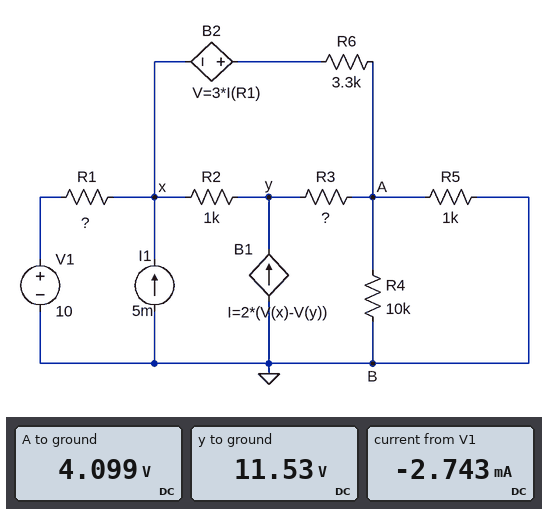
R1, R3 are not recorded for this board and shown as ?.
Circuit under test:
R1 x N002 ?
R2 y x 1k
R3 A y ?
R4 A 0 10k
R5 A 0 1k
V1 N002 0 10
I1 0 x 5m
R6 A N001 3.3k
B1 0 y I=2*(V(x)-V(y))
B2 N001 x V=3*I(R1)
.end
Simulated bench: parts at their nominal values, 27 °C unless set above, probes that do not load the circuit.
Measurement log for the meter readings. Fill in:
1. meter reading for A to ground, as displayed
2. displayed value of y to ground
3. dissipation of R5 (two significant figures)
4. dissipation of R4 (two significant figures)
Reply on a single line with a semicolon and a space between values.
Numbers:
4.099 V; 11.53 V; 17 mW; 1.7 mW
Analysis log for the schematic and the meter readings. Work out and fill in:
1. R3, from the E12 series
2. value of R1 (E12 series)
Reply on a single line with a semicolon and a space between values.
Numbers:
3.3 kΩ; 560 Ω
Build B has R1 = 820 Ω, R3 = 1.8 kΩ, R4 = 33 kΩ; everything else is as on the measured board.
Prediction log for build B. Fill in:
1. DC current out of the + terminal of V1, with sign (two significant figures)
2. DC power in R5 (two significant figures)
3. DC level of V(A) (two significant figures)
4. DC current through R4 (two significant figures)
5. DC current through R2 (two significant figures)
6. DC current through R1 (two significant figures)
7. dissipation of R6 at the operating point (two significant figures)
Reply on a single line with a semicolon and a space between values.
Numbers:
-2.9 mA; 32 mW; 5.6 V; 170 µA; 1.9 µA; 2.9 mA; 14 mW
